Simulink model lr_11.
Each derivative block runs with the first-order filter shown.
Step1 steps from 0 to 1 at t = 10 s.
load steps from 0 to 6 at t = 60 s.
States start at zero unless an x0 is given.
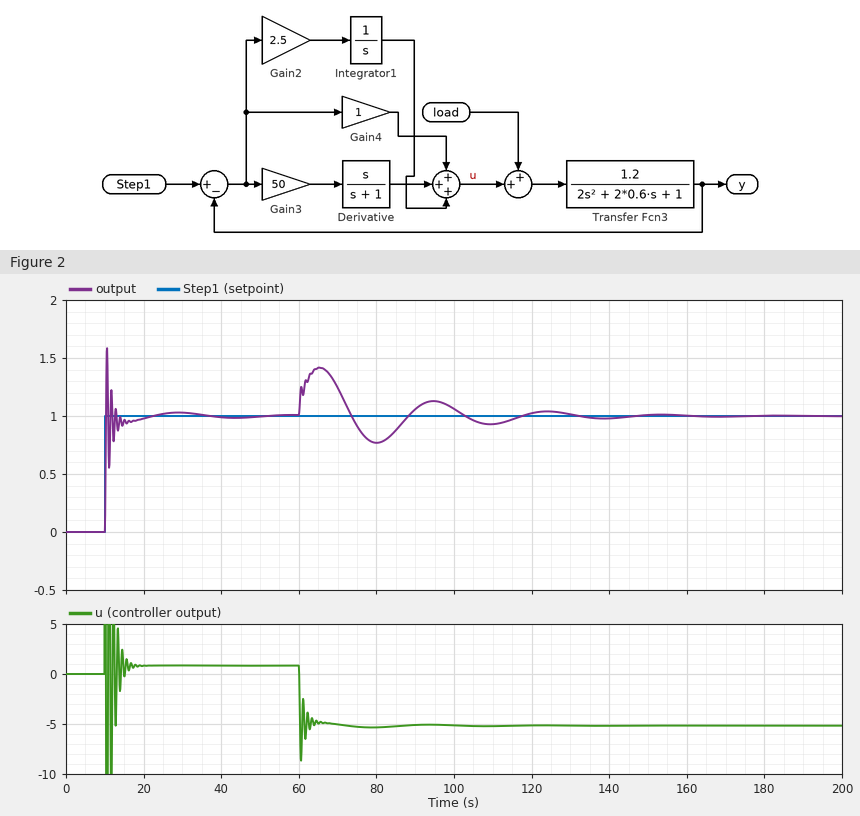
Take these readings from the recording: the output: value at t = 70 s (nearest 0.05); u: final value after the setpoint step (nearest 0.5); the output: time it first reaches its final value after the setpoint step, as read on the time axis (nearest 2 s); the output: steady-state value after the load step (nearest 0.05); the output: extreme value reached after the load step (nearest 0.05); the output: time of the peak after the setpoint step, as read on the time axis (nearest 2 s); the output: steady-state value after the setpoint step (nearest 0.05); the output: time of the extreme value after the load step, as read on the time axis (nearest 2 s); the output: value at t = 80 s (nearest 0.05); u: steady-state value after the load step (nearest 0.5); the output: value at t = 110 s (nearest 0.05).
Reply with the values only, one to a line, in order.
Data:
1.25
1.0
10 s
1.00
1.40
10 s
1.00
66 s
0.75
-5.0
0.95
